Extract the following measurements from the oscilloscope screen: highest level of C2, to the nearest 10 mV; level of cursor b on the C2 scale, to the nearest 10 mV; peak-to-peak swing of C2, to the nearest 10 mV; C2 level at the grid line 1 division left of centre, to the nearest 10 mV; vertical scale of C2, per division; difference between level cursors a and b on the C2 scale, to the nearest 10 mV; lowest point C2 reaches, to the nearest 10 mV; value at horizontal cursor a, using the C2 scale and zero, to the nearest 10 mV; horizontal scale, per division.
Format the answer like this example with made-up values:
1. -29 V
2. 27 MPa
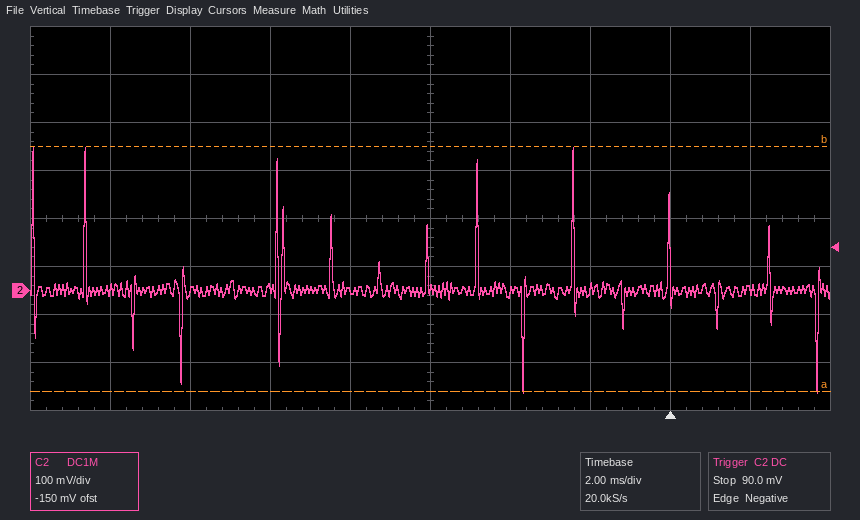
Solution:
1. 300 mV
2. 300 mV
3. 510 mV
4. 0 mV
5. 100 mV
6. 510 mV
7. -210 mV
8. -210 mV
9. 2 ms
